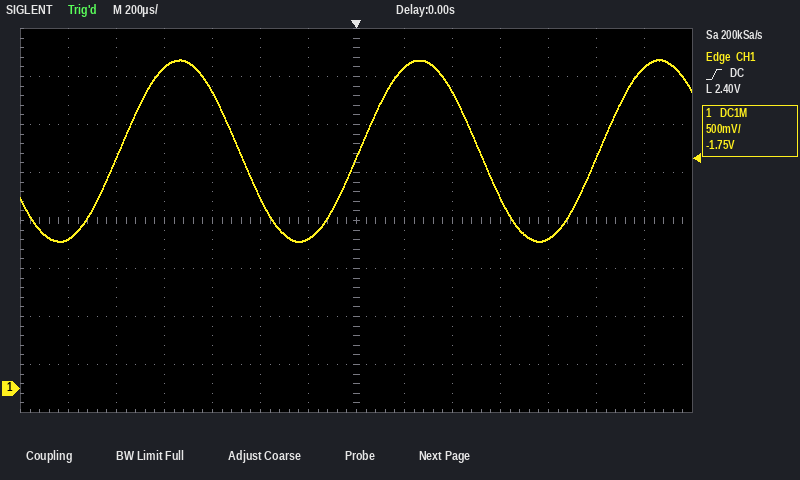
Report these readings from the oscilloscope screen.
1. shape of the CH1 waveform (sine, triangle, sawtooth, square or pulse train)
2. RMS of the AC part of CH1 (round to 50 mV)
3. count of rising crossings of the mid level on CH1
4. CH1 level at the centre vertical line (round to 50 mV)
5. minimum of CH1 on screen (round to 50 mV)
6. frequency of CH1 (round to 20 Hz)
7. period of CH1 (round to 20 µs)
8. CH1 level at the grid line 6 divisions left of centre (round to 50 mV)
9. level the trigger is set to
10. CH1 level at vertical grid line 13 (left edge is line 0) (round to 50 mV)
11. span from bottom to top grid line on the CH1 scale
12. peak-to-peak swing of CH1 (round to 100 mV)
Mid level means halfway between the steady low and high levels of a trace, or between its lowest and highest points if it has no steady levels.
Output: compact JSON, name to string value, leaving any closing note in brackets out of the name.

{"shape of the CH1 waveform": "sine", "RMS of the AC part of CH1": "650 mV", "count of rising crossings of the mid level on CH1": "3", "CH1 level at the centre vertical line": "2.40 V", "minimum of CH1 on screen": "1.55 V", "frequency of CH1": "1.00 kHz", "period of CH1": "1.00 ms", "CH1 level at the grid line 6 divisions left of centre": "1.55 V", "level the trigger is set to": "2.40 V", "CH1 level at vertical grid line 13 (left edge is line 0)": "3.35 V", "span from bottom to top grid line on the CH1 scale": "4 V", "peak-to-peak swing of CH1": "1.90 V"}
